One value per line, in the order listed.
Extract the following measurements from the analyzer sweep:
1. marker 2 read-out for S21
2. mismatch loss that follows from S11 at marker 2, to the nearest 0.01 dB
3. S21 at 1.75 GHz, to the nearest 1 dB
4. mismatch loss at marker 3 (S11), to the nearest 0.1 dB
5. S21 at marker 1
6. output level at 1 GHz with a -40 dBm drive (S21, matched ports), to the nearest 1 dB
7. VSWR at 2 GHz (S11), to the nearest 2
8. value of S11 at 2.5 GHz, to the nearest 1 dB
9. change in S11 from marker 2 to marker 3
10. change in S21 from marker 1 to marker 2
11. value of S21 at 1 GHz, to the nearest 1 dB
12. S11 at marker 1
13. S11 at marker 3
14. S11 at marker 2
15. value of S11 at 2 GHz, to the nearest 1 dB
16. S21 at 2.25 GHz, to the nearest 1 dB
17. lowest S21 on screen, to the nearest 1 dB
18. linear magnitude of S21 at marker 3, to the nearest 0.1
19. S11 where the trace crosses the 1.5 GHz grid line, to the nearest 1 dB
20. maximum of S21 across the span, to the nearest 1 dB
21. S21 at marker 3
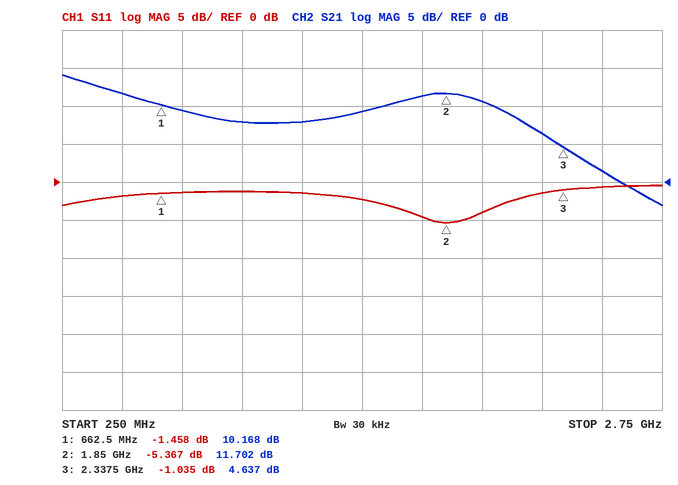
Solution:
11.702 dB
1.49 dB
11 dB
6.7 dB
10.168 dB
-32 dBm
4
-1 dB
4.332 dB
1.534 dB
8 dB
-1.458 dB
-1.035 dB
-5.367 dB
-4 dB
6 dB
-3 dB
1.7
-2 dB
14 dB
4.637 dB
